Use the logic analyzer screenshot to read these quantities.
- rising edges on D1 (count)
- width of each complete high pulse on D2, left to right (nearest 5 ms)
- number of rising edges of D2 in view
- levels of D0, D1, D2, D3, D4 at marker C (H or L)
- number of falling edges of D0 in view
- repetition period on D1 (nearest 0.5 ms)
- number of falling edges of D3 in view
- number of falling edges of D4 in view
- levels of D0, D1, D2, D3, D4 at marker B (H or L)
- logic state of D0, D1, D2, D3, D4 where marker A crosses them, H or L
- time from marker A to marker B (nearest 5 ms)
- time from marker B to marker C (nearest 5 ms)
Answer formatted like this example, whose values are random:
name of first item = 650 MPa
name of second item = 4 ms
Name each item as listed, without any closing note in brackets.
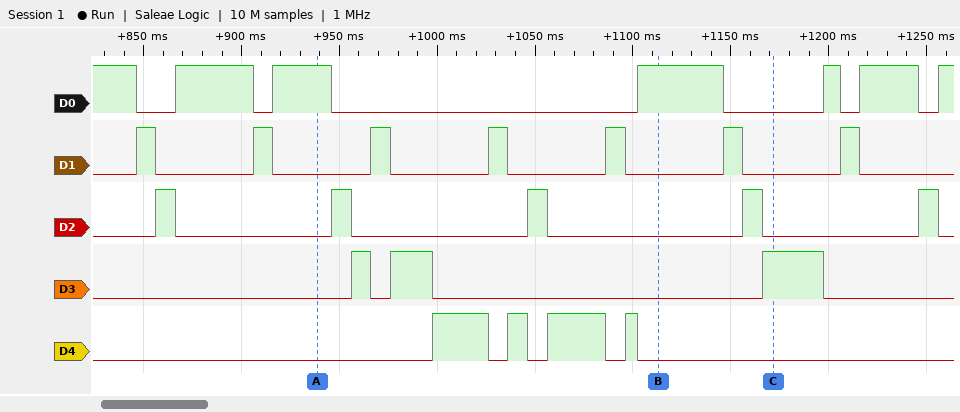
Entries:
rising edges on D1 = 7
width of each complete high pulse on D2, left to right = 10 ms, 10 ms, 10 ms, 10 ms, 10 ms
number of rising edges of D2 in view = 5
levels of D0, D1, D2, D3, D4 at marker C = D0=L, D1=L, D2=L, D3=H, D4=L
number of falling edges of D0 in view = 6
repetition period on D1 = 60 ms
number of falling edges of D3 in view = 3
number of falling edges of D4 in view = 4
levels of D0, D1, D2, D3, D4 at marker B = D0=H, D1=L, D2=L, D3=L, D4=L
logic state of D0, D1, D2, D3, D4 where marker A crosses them, H or L = D0=H, D1=L, D2=L, D3=L, D4=L
time from marker A to marker B = 175 ms
time from marker B to marker C = 60 ms
